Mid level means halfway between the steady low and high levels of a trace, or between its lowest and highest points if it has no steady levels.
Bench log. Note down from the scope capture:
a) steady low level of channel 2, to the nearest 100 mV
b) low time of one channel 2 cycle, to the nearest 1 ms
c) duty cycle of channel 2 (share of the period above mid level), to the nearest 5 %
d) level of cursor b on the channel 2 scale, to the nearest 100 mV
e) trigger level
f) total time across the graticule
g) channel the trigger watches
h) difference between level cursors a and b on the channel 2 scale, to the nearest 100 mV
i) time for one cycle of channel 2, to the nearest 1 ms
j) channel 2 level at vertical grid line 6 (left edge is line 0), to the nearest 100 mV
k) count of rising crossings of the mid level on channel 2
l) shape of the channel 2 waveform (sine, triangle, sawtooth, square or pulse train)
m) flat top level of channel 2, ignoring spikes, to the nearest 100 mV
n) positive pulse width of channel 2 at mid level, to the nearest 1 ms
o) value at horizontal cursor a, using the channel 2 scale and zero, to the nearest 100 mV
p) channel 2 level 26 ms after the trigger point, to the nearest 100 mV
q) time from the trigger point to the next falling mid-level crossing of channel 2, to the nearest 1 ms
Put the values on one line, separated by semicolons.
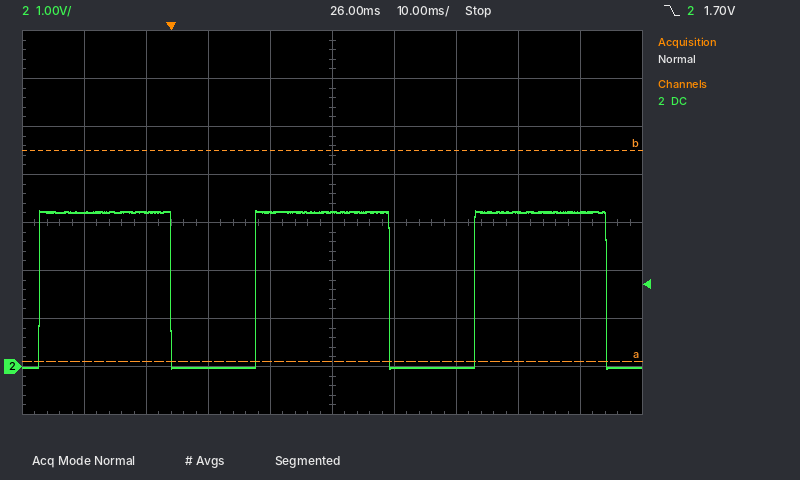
0.0 V; 14 ms; 60 %; 4.5 V; 1.70 V; 100 ms; channel 2; 4.4 V; 35 ms; 0.0 V; 3; pulse train; 3.2 V; 21 ms; 100 mV; 3.2 V; 35 ms
